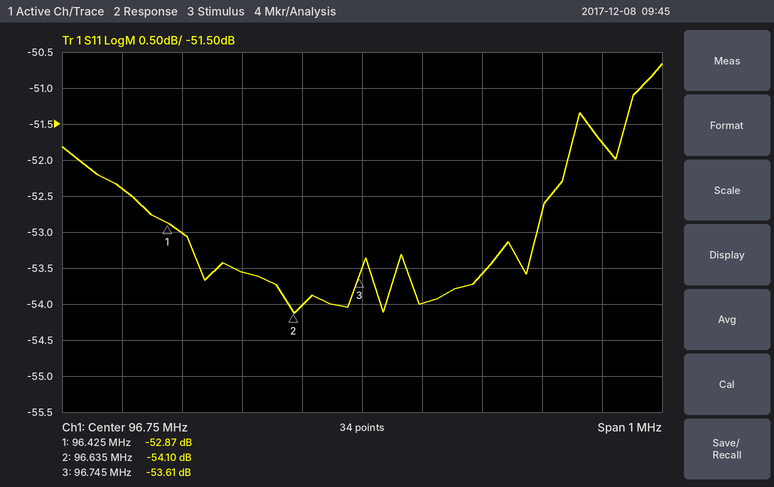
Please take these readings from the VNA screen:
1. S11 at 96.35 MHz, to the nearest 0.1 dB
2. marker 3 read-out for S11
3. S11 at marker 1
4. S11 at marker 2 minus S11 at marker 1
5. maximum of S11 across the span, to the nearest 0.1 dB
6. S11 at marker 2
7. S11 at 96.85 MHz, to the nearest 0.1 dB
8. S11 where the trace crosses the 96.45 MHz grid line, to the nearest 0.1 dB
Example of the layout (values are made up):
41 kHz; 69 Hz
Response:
-52.4 dB; -53.61 dB; -52.87 dB; -1.23 dB; -50.7 dB; -54.10 dB; -54.0 dB; -53.0 dB
